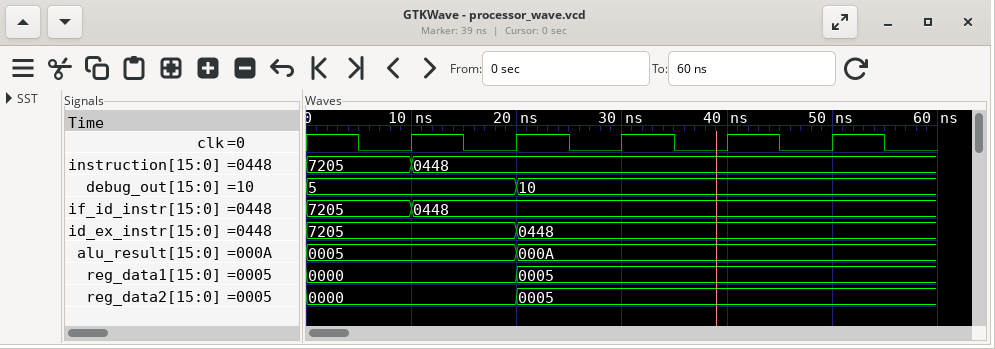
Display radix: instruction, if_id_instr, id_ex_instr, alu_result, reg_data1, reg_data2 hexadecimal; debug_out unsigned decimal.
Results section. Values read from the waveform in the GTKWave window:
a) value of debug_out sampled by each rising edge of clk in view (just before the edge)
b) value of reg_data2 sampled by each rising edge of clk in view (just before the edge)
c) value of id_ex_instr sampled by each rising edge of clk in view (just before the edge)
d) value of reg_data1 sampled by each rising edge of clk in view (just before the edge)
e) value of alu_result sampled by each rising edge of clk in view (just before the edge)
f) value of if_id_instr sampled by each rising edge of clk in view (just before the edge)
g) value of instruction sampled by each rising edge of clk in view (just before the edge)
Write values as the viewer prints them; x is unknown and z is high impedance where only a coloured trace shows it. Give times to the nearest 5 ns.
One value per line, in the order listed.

5, 5, 10, 10, 10
0000, 0000, 0005, 0005, 0005
7205, 7205, 0448, 0448, 0448
0000, 0000, 0005, 0005, 0005
0005, 0005, 000A, 000A, 000A
7205, 0448, 0448, 0448, 0448
7205, 0448, 0448, 0448, 0448
